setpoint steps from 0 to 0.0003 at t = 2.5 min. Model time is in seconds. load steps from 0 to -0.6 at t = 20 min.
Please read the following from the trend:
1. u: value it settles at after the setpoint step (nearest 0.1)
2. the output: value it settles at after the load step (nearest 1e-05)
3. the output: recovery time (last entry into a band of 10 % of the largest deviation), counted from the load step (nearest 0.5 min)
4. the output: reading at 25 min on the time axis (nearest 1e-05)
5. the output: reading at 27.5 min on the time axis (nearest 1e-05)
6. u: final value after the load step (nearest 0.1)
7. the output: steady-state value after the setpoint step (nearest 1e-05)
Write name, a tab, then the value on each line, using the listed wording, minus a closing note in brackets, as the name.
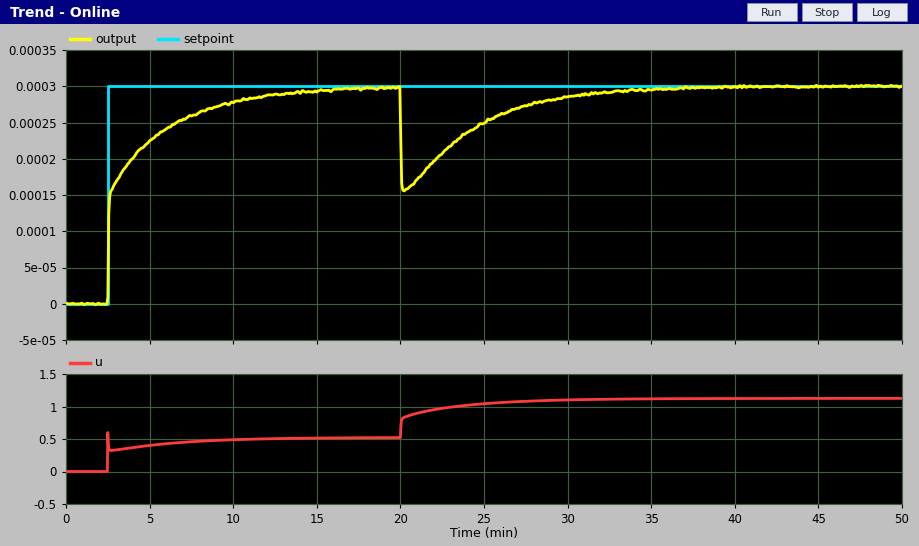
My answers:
u: value it settles at after the setpoint step	0.5
the output: value it settles at after the load step	0.00030
the output: recovery time (last entry into a band of 10 % of the largest deviation), counted from the load step	10.0 min
the output: reading at 25 min on the time axis	0.00025
the output: reading at 27.5 min on the time axis	0.00027
u: final value after the load step	1.1
the output: steady-state value after the setpoint step	0.00030
